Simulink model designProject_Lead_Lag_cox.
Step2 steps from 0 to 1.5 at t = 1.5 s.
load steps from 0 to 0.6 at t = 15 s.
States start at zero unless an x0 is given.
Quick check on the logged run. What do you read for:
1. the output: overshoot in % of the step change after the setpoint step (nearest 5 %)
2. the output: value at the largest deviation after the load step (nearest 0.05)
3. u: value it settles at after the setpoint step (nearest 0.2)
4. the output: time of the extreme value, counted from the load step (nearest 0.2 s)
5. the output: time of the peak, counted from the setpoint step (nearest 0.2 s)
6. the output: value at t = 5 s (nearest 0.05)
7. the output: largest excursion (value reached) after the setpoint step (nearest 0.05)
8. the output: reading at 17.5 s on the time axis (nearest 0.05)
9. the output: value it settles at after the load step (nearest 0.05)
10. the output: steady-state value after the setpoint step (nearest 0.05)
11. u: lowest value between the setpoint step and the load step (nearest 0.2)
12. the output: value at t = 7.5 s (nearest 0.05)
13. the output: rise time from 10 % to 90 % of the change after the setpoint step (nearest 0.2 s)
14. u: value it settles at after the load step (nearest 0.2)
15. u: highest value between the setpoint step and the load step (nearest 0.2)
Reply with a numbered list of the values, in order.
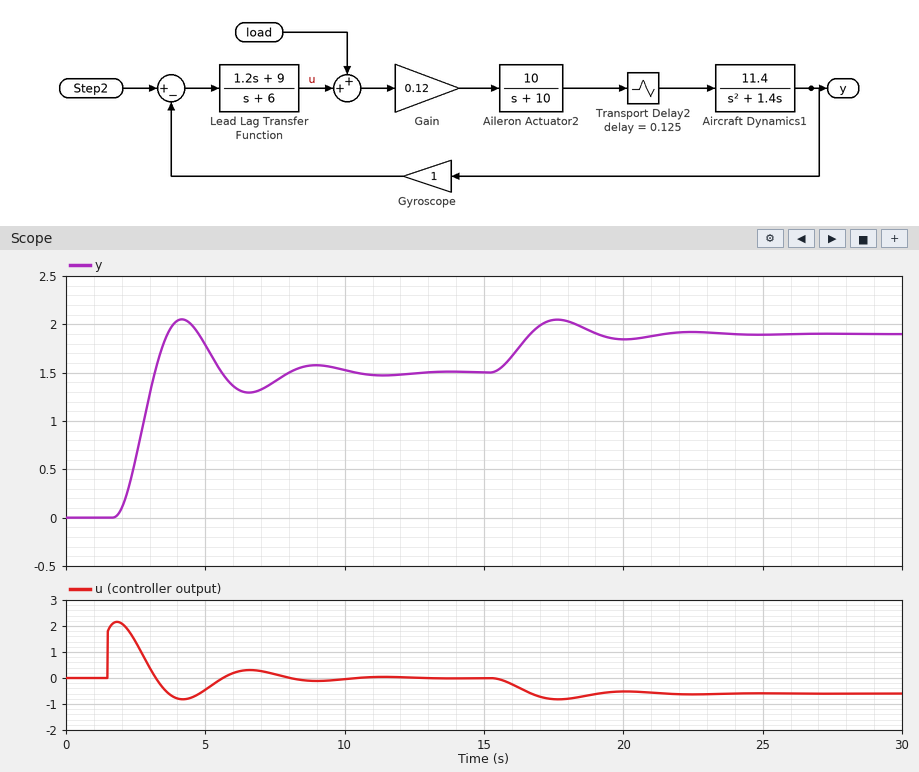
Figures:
1. 35 %
2. 2.05
3. 0.0
4. 2.6 s
5. 2.6 s
6. 1.80
7. 2.05
8. 2.05
9. 1.90
10. 1.50
11. -0.8
12. 1.40
13. 1.0 s
14. -0.6
15. 2.2
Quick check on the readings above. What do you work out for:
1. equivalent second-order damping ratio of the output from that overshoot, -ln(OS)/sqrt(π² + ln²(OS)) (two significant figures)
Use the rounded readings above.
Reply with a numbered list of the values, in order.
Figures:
1. 0.32
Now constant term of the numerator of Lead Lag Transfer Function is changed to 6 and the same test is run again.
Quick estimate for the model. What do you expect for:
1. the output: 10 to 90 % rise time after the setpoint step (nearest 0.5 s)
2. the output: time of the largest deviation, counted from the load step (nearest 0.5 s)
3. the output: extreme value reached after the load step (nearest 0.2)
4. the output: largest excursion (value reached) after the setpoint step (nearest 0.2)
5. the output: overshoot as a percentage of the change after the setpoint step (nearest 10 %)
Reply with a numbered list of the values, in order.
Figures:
1. 1.5 s
2. 3.5 s
3. 2.2
4. 1.8
5. 20 %
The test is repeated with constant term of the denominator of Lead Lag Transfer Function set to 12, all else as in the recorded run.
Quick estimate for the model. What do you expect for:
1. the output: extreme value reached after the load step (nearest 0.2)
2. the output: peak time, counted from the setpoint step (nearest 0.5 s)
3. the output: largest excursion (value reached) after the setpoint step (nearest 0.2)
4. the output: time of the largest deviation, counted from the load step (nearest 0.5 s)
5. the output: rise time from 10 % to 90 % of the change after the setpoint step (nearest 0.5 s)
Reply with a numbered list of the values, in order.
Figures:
1. 2.4
2. 4.0 s
3. 1.6
4. 4.0 s
5. 2.0 s
